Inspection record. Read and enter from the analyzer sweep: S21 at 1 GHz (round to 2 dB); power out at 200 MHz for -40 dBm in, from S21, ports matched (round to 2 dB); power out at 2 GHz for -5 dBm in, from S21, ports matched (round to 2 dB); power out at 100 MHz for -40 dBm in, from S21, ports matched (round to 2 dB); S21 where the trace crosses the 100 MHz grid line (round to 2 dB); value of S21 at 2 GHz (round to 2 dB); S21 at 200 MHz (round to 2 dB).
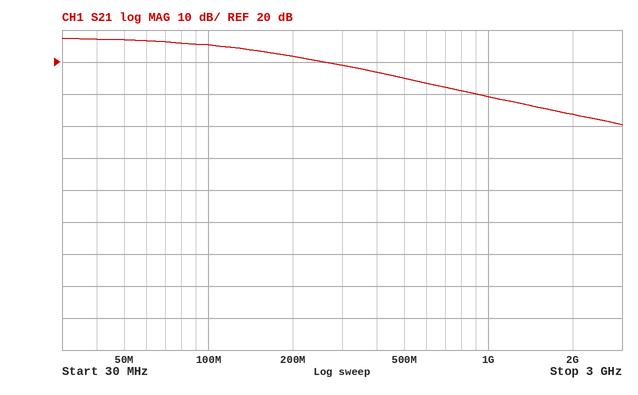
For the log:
10 dB
-18 dBm
-2 dBm
-14 dBm
26 dB
4 dB
22 dB
